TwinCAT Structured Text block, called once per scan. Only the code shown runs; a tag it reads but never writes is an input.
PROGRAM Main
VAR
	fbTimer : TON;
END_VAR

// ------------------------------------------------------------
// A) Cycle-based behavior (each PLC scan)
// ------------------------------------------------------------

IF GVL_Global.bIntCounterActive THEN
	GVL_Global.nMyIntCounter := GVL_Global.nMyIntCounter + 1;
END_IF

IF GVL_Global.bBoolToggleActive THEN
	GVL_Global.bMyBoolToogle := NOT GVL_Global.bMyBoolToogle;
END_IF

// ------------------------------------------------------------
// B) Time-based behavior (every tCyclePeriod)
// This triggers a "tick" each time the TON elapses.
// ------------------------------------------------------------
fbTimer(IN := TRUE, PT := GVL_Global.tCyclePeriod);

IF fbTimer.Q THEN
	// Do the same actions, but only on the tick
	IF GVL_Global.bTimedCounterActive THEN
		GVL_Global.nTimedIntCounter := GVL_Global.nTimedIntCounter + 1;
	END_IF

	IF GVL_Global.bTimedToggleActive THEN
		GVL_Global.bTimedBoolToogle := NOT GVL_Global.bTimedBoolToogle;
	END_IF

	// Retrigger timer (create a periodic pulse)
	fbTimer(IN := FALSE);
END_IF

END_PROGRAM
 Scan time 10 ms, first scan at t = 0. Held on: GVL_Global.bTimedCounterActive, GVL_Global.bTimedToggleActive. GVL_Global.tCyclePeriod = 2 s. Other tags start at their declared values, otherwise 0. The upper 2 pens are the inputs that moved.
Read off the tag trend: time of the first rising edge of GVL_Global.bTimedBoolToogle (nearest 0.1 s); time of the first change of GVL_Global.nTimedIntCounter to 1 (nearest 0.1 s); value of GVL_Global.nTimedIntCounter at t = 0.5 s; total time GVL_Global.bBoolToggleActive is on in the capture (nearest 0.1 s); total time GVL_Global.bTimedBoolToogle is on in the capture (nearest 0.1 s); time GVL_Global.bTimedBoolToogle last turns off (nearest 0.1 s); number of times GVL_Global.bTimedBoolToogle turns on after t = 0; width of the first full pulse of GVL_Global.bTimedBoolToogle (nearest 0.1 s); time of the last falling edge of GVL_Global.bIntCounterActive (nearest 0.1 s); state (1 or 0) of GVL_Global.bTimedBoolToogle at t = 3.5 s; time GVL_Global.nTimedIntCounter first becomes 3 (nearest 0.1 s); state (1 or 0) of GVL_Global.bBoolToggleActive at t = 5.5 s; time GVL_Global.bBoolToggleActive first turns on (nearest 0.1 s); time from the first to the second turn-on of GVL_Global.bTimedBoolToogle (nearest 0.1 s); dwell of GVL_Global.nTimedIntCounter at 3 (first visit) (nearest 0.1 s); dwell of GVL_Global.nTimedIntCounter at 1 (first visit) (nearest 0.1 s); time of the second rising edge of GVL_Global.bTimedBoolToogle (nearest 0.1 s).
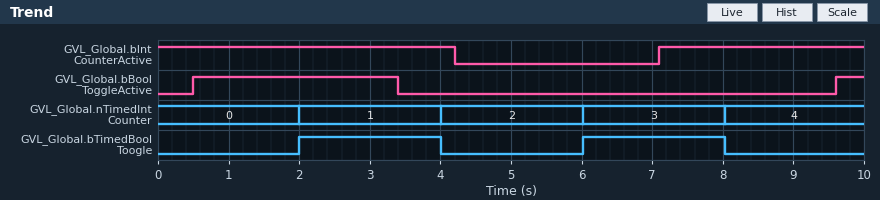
2.0 s
2.0 s
0
3.3 s
4.0 s
8.0 s
2
2.0 s
4.2 s
1
6.0 s
0
0.5 s
4.0 s
2.0 s
2.0 s
6.0 s
